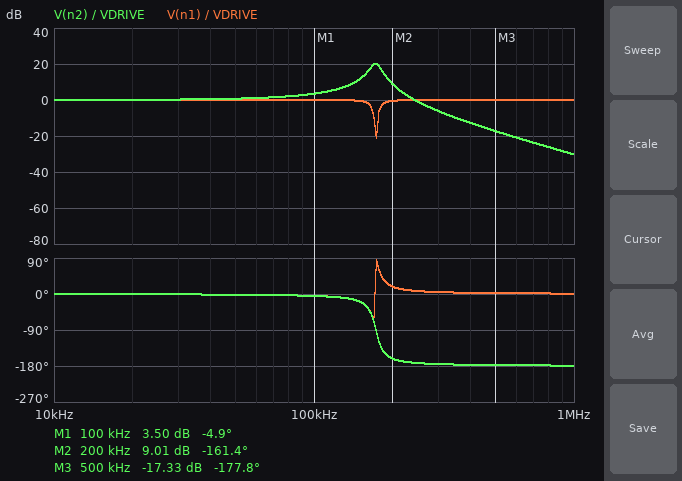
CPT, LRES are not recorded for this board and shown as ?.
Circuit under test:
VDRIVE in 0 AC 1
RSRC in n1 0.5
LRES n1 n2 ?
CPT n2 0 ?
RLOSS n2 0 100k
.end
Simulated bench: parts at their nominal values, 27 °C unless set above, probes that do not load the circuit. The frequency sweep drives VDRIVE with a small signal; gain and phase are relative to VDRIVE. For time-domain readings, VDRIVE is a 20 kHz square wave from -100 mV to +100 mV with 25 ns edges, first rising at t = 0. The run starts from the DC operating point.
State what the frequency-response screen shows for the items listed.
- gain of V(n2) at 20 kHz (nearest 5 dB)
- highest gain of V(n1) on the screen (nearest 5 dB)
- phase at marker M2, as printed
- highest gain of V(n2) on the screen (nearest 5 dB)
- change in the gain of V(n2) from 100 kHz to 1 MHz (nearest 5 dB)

0 dB
0 dB
-161.4 deg
20 dB
-35 dB
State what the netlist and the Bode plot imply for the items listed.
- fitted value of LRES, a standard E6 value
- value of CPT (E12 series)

4.7 µH
180 nF
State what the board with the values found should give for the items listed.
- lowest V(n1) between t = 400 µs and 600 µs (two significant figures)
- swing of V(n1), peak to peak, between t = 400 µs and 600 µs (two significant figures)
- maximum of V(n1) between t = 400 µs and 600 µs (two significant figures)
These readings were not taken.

-120 mV
230 mV
120 mV
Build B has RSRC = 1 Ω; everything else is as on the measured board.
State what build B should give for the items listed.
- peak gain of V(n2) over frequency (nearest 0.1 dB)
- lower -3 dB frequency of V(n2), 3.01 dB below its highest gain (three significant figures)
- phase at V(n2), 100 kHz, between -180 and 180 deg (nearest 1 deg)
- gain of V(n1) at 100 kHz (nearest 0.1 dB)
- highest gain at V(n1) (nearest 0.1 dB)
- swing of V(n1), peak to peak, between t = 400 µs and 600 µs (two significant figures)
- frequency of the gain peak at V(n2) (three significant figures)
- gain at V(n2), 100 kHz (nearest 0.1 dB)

14.2 dB
153 kHz
-10 deg
-0.1 dB
0 dB
250 mV
171 kHz
3.4 dB
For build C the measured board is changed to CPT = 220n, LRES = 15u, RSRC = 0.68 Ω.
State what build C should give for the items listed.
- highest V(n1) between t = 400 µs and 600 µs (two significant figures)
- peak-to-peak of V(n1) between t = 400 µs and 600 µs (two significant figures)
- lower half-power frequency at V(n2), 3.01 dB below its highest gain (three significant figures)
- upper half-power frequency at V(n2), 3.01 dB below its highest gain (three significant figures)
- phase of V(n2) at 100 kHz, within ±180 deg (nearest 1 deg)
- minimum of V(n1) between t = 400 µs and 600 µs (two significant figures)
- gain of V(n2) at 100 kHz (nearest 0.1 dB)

110 mV
220 mV
83.8 kHz
91.0 kHz
-163 deg
-110 mV
10.0 dB
